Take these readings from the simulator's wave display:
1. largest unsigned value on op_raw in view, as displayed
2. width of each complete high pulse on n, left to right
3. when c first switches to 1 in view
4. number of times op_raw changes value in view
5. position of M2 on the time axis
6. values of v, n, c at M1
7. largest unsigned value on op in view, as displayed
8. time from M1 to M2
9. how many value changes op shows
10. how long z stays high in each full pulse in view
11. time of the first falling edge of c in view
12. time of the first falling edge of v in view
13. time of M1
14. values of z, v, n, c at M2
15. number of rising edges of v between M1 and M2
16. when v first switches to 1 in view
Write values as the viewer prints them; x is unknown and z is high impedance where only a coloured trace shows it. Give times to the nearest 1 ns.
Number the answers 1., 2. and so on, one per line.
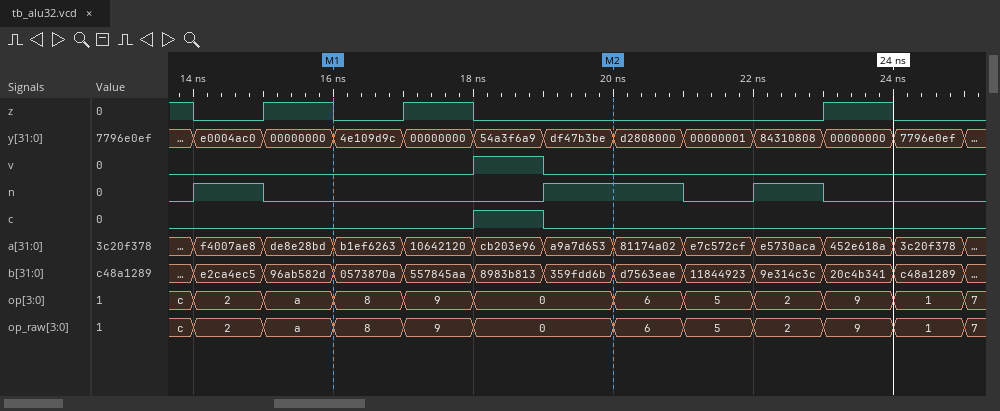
1. c
2. 1 ns, 2 ns, 1 ns
3. 18 ns
4. 11
5. 20 ns
6. v=0, n=0, c=0
7. c
8. 4 ns
9. 11
10. 1 ns, 1 ns, 1 ns
11. 19 ns
12. 19 ns
13. 16 ns
14. z=0, v=0, n=1, c=0
15. 1
16. 18 ns
